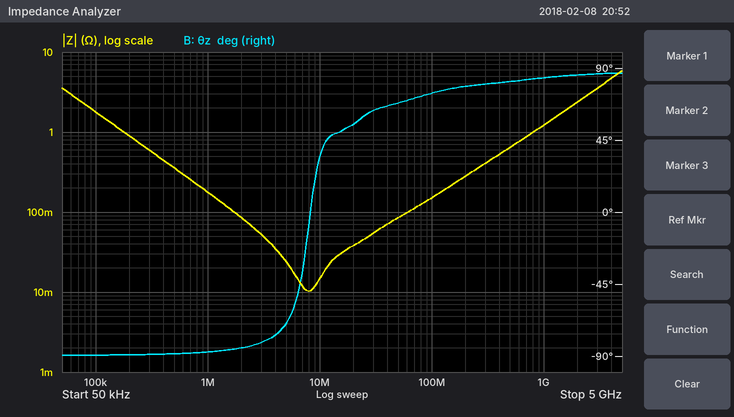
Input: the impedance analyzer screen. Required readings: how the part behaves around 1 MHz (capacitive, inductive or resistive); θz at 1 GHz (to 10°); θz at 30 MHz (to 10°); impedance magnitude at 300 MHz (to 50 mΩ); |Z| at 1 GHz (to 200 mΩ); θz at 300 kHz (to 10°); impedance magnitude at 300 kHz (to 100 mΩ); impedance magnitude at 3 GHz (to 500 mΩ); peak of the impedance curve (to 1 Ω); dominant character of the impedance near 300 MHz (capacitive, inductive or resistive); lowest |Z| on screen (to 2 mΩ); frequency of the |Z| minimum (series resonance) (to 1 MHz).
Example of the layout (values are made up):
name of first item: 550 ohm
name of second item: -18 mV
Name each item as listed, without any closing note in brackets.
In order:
how the part behaves around 1 MHz: capacitive
θz at 1 GHz: 80°
θz at 30 MHz: 60°
impedance magnitude at 300 MHz: 400 mΩ
|Z| at 1 GHz: 1.2 Ω
θz at 300 kHz: -90°
impedance magnitude at 300 kHz: 600 mΩ
impedance magnitude at 3 GHz: 3.5 Ω
peak of the impedance curve: 6 Ω
dominant character of the impedance near 300 MHz: inductive
lowest |Z| on screen: 10 mΩ
frequency of the |Z| minimum (series resonance): 8 MHz
